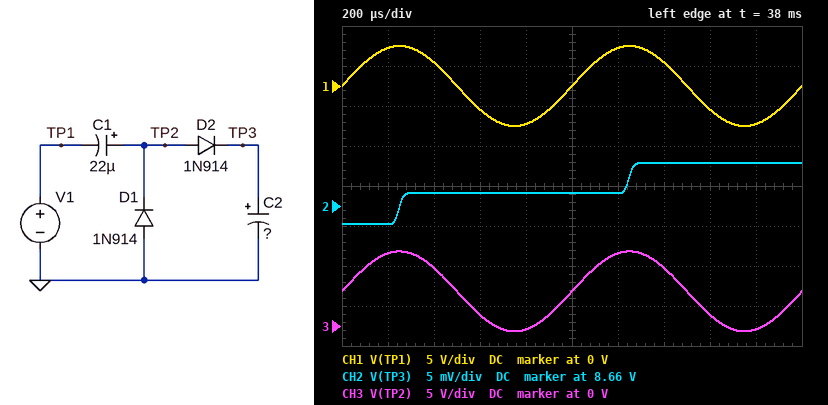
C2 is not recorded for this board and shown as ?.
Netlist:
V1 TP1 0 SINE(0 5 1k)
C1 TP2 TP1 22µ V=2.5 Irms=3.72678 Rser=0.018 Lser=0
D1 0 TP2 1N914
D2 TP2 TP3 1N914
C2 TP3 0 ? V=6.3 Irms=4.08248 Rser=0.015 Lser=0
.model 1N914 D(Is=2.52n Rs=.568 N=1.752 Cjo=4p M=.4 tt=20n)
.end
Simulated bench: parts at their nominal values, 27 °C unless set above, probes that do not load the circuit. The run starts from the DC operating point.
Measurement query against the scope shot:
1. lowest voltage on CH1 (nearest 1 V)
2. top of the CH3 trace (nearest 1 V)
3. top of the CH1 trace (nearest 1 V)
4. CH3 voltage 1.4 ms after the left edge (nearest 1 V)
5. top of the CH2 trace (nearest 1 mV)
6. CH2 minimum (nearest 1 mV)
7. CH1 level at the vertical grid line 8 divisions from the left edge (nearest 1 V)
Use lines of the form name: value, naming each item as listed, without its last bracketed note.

lowest voltage on CH1: -5 V
top of the CH3 trace: 9 V
top of the CH1 trace: 5 V
CH3 voltage 1.4 ms after the left edge: 7 V
top of the CH2 trace: 8.665 V
CH2 minimum: 8.658 V
CH1 level at the vertical grid line 8 divisions from the left edge: -3 V
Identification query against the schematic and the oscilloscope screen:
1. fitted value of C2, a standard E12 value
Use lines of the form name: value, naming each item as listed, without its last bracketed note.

fitted value of C2, a standard E12 value: 56 µF
